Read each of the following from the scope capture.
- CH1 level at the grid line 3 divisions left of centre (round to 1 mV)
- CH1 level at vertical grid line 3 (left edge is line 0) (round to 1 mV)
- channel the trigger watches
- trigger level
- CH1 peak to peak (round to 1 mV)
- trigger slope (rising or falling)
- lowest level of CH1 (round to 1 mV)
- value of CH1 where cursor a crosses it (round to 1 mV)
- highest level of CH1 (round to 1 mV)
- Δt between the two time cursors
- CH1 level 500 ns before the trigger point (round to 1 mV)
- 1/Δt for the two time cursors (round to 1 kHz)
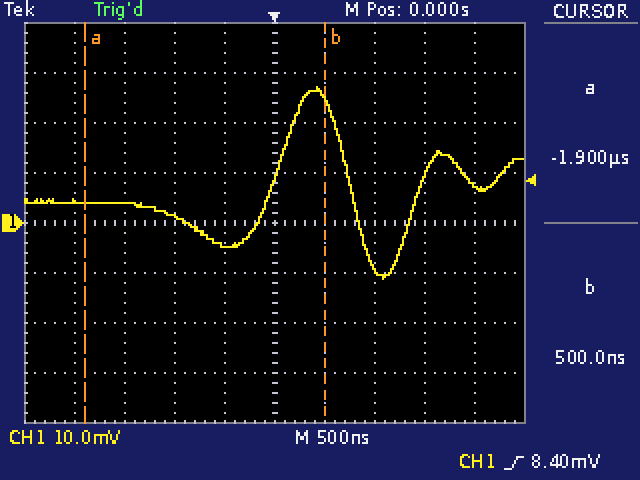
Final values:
4 mV
1 mV
CH1
8.40 mV
38 mV
rising
-11 mV
4 mV
27 mV
2.40 µs
-4 mV
417 kHz
